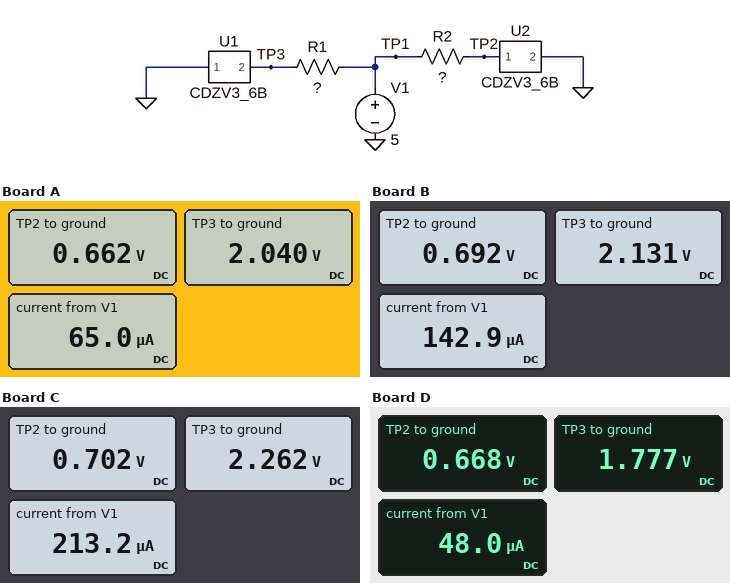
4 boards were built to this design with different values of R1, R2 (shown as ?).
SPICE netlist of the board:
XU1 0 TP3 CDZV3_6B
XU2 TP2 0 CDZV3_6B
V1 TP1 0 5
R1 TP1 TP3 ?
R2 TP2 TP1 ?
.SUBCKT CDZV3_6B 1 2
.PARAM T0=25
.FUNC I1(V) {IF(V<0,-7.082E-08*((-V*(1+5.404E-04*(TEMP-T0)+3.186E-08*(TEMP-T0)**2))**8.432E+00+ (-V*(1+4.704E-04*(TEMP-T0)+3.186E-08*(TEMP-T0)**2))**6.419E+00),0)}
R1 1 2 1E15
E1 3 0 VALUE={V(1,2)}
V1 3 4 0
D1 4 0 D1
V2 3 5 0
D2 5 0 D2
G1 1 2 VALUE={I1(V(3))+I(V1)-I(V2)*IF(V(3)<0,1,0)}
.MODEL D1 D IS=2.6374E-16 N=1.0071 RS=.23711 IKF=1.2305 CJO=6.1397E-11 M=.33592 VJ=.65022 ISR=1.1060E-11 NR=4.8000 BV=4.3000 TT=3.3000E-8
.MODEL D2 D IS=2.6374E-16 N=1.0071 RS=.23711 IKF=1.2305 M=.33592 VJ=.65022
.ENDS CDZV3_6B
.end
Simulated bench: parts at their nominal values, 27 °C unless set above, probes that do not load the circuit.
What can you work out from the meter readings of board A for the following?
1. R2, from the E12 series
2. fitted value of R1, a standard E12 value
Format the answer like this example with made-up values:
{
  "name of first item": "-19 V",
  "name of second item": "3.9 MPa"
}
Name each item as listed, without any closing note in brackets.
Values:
{
  "R2, from the E12 series": "150 kΩ",
  "fitted value of R1, a standard E12 value": "82 kΩ"
}
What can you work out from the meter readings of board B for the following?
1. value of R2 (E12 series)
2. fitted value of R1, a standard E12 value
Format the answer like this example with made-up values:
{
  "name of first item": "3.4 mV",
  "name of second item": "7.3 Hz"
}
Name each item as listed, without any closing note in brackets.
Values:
{
  "value of R2": "47 kΩ",
  "fitted value of R1, a standard E12 value": "56 kΩ"
}
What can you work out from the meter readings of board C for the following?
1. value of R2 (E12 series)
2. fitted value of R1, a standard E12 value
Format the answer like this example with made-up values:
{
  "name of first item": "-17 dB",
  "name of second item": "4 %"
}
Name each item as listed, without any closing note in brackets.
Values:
{
  "value of R2": "33 kΩ",
  "fitted value of R1, a standard E12 value": "33 kΩ"
}
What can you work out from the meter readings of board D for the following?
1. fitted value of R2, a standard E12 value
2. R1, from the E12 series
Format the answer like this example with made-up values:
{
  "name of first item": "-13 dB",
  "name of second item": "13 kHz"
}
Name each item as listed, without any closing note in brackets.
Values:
{
  "fitted value of R2, a standard E12 value": "120 kΩ",
  "R1, from the E12 series": "270 kΩ"
}
